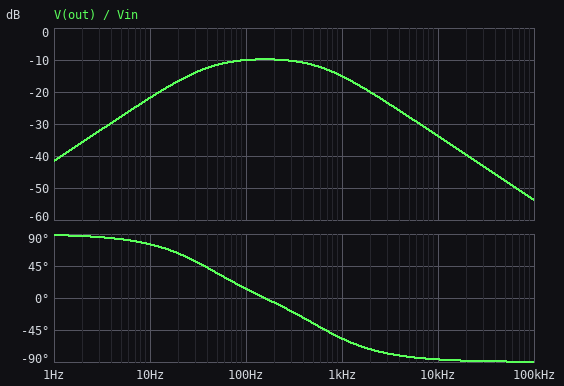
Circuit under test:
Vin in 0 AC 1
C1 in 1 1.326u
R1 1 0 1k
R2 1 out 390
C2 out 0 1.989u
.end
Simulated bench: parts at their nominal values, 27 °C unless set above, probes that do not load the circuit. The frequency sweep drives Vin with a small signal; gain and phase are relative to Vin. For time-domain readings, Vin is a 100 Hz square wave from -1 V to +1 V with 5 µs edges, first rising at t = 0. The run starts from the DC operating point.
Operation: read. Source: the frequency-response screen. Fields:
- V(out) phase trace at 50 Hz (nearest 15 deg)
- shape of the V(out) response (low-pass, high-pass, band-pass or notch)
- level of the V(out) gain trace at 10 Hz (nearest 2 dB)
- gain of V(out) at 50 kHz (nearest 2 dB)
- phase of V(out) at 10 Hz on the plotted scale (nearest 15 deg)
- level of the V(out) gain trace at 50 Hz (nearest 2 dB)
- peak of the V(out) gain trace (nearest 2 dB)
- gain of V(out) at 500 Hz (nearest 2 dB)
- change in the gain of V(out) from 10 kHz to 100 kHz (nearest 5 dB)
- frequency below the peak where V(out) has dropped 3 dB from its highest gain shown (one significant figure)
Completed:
30 deg
band-pass
-22 dB
-48 dB
75 deg
-12 dB
-10 dB
-12 dB
-20 dB
40 Hz
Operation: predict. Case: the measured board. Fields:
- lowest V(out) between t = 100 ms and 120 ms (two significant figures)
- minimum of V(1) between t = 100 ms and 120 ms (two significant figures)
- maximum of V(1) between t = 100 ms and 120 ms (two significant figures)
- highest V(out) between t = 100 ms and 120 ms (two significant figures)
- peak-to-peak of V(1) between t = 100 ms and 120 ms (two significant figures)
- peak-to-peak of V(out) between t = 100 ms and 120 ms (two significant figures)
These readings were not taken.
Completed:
-440 mV
-1.9 V
1.9 V
440 mV
3.7 V
880 mV
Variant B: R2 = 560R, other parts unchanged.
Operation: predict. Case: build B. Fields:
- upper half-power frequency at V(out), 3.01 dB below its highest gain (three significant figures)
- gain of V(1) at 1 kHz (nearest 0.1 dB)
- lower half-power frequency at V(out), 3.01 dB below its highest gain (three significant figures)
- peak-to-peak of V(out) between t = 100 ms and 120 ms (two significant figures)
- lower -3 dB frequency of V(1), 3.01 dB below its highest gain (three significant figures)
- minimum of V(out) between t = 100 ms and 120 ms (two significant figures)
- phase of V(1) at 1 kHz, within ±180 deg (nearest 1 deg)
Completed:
511 Hz
-0.7 dB
33.6 Hz
780 mV
393 Hz
-390 mV
18 deg
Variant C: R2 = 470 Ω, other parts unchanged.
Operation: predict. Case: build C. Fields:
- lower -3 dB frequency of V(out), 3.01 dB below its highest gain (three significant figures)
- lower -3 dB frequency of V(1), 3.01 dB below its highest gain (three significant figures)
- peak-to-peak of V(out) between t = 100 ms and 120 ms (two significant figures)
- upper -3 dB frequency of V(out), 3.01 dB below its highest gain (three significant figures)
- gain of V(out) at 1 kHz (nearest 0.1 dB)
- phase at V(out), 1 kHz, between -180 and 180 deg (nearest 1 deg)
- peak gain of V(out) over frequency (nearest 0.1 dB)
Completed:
35.2 Hz
448 Hz
830 mV
581 Hz
-16.4 dB
-61 deg
-10.1 dB
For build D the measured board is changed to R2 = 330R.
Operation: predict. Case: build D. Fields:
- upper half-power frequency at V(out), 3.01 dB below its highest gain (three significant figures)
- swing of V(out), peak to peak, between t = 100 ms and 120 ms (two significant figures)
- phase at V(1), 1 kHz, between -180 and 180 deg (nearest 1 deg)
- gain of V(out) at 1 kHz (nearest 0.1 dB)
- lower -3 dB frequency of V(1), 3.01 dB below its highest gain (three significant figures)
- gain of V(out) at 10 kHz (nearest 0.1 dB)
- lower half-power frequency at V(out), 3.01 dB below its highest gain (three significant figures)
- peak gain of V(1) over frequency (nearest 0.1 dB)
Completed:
764 Hz
920 mV
23 deg
-14.0 dB
595 Hz
-32.3 dB
38.1 Hz
0 dB
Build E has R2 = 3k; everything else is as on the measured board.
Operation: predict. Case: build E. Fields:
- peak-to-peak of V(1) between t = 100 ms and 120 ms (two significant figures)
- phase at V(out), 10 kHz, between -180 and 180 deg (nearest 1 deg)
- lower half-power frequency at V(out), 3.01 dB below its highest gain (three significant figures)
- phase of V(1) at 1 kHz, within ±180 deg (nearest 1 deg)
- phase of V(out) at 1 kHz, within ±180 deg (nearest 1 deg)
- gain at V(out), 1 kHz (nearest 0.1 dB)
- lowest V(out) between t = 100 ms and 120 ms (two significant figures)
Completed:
3.9 V
-89 deg
15.8 Hz
9 deg
-79 deg
-31.6 dB
-150 mV
